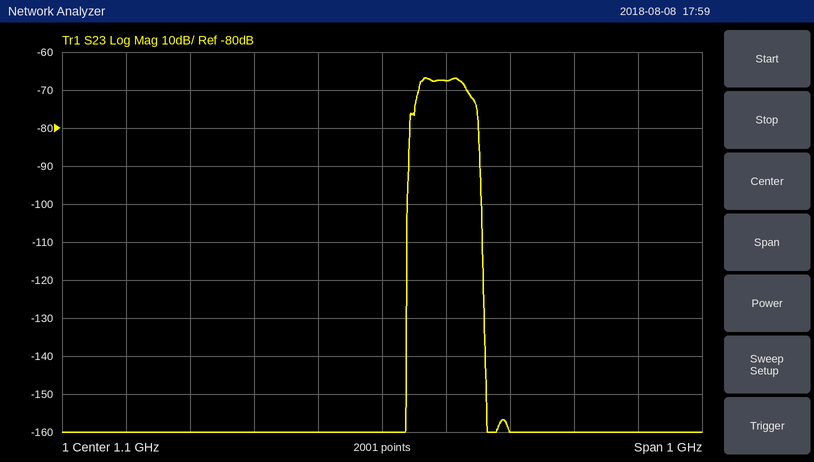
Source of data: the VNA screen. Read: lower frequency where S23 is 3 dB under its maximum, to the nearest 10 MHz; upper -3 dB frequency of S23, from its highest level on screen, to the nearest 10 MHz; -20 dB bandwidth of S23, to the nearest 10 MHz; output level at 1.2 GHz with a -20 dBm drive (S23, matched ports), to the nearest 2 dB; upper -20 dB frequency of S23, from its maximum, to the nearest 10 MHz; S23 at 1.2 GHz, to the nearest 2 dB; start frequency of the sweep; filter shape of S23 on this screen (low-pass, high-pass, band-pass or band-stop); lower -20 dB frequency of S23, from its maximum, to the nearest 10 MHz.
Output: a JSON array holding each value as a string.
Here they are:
["1.16 GHz", "1.23 GHz", "110 MHz", "-88 dBm", "1.25 GHz", "-68 dB", "600 MHz", "band-pass", "1.14 GHz"]
